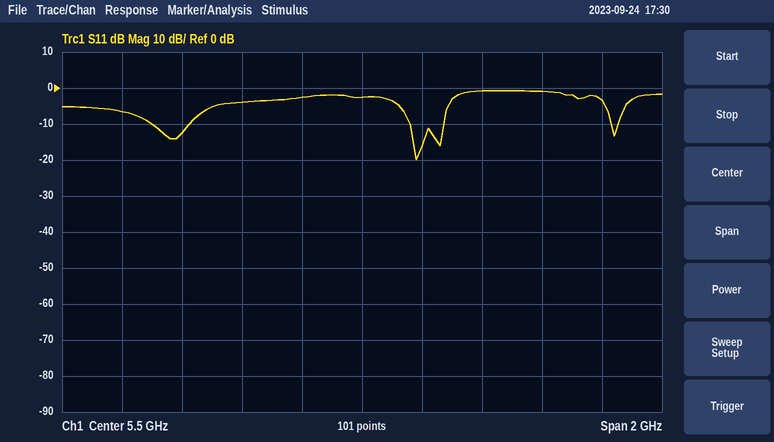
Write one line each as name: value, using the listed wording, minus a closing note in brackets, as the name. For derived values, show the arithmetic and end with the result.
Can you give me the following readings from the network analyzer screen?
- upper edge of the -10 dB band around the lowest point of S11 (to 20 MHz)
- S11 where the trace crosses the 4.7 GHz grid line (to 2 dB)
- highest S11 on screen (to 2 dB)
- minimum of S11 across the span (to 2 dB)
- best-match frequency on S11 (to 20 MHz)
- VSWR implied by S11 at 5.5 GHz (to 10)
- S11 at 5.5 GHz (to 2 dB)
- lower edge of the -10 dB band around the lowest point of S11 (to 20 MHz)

upper edge of the -10 dB band around the lowest point of S11: 5.78 GHz
S11 where the trace crosses the 4.7 GHz grid line: -6 dB
highest S11 on screen: 0 dB
minimum of S11 across the span: -20 dB
best-match frequency on S11: 5.68 GHz
VSWR implied by S11 at 5.5 GHz: |Γ| = 10^(-2/20) = 0.7943; VSWR = (1 + 0.7943)/(1 − 0.7943) ≈ 8.72, so 10 to the nearest 10
S11 at 5.5 GHz: -2 dB
lower edge of the -10 dB band around the lowest point of S11: 5.66 GHz
